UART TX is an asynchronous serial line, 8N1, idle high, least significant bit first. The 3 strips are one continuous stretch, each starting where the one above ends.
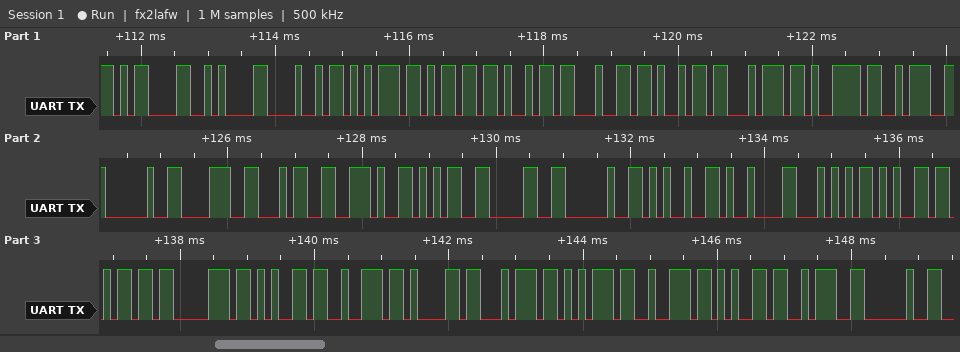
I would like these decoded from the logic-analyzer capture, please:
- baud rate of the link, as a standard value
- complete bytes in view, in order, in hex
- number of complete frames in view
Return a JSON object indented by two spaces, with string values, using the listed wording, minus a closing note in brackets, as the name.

{
  "baud rate of the link, as a standard value": "9600 baud",
  "complete bytes in view, in order, in hex": "0D 0A 48 75 6D 69 64 69 74 79 3A 20 38 34 2E 35 30 20 25 09 54 65 6D 70 65 72 61 74 75 72 65 3A 20",
  "number of complete frames in view": "33"
}
